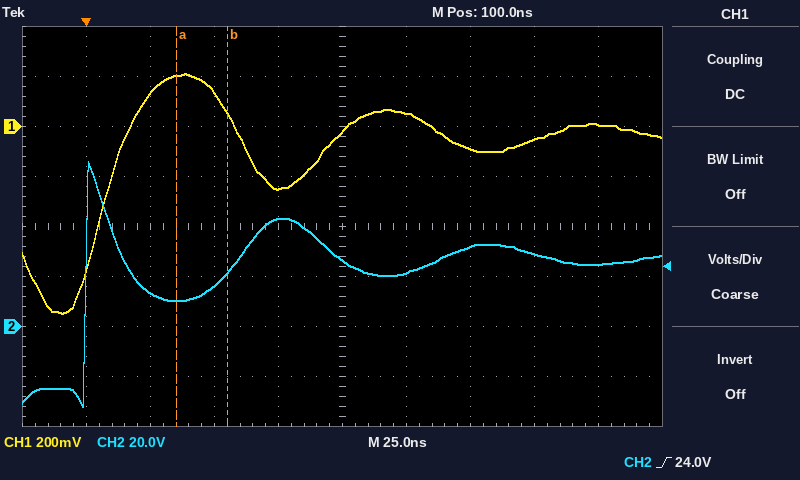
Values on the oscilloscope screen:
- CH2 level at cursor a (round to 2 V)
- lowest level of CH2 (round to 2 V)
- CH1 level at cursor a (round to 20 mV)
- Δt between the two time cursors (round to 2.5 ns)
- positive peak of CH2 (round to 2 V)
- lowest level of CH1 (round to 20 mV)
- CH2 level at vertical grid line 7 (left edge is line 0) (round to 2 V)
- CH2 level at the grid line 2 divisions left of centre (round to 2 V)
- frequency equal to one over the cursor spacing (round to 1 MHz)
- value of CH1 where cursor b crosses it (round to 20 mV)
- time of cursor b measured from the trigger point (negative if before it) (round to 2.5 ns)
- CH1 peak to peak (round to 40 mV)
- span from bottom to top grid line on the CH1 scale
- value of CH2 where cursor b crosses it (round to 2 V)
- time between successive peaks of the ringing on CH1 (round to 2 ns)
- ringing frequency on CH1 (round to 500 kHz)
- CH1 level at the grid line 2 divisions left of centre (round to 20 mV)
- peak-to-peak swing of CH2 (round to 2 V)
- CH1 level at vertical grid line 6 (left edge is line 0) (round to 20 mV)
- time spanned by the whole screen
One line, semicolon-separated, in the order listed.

10 V; -32 V; 200 mV; 20.0 ns; 66 V; -740 mV; 32 V; 16 V; 50 MHz; 60 mV; +55.0 ns; 960 mV; 1.6 V; 22 V; 80 ns; 12.5 MHz; 140 mV; 98 V; 60 mV; 250 ns
